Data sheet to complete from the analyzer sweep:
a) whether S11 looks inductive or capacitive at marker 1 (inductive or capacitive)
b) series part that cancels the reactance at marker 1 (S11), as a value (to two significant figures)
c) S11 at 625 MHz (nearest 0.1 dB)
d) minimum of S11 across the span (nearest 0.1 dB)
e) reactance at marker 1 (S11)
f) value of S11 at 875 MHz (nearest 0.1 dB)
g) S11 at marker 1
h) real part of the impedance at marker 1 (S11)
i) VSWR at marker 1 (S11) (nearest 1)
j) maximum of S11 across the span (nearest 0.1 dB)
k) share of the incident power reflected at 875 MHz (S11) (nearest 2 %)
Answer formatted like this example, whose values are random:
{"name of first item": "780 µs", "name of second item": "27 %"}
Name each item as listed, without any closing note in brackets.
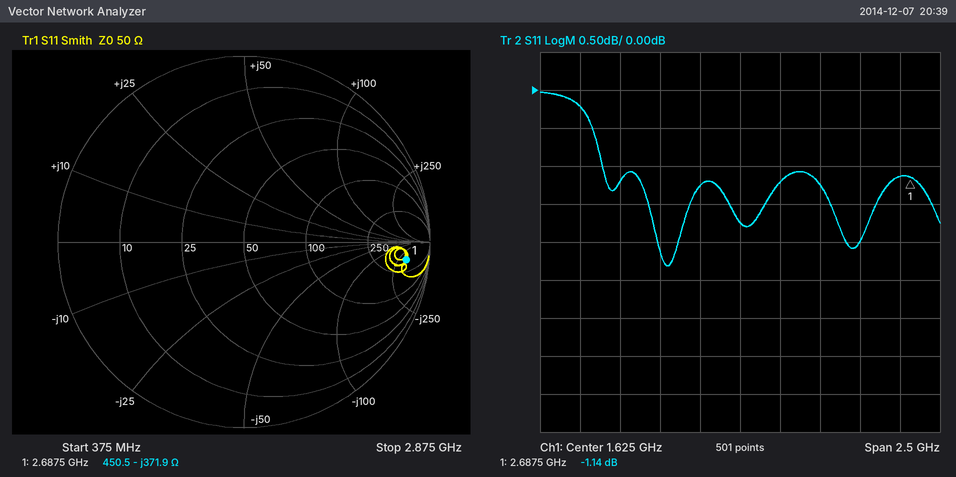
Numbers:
{"whether S11 looks inductive or capacitive at marker 1": "capacitive", "series part that cancels the reactance at marker 1 (S11), as a value": "22 nH", "S11 at 625 MHz": "-0.2 dB", "minimum of S11 across the span": "-2.3 dB", "reactance at marker 1": "-371.9 Ω", "value of S11 at 875 MHz": "-1.2 dB", "S11 at marker 1": "-1.14 dB", "real part of the impedance at marker 1": "450.5 Ω", "VSWR at marker 1 (S11)": "15", "maximum of S11 across the span": "0.0 dB", "share of the incident power reflected at 875 MHz (S11)": "76 %"}
